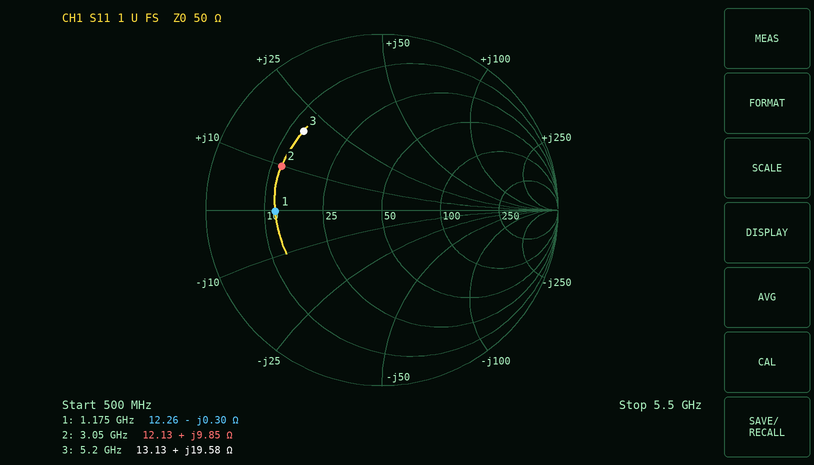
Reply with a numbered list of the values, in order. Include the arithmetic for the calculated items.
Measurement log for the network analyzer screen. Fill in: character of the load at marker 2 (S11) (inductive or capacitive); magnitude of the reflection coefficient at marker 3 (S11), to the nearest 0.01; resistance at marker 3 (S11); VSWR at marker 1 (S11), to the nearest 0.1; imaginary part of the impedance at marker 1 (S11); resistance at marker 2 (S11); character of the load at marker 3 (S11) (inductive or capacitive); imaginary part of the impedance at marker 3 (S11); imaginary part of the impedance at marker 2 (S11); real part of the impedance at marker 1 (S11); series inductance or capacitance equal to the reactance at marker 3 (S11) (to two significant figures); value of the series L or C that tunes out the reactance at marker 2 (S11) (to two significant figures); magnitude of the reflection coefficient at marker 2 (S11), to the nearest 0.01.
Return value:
1. inductive
2. 0.63
3. 13.13 Ω
4. 4.1
5. -0.30 Ω
6. 12.13 Ω
7. inductive
8. +19.58 Ω
9. +9.85 Ω
10. 12.26 Ω
11. L = 19.58 Ω/(2π × 5.2 GHz) ≈ 599 pH, so 600 pH to two significant figures
12. C = 1/(2π × 3.05 GHz × 9.85 Ω) ≈ 5.3 pF
13. 0.62
